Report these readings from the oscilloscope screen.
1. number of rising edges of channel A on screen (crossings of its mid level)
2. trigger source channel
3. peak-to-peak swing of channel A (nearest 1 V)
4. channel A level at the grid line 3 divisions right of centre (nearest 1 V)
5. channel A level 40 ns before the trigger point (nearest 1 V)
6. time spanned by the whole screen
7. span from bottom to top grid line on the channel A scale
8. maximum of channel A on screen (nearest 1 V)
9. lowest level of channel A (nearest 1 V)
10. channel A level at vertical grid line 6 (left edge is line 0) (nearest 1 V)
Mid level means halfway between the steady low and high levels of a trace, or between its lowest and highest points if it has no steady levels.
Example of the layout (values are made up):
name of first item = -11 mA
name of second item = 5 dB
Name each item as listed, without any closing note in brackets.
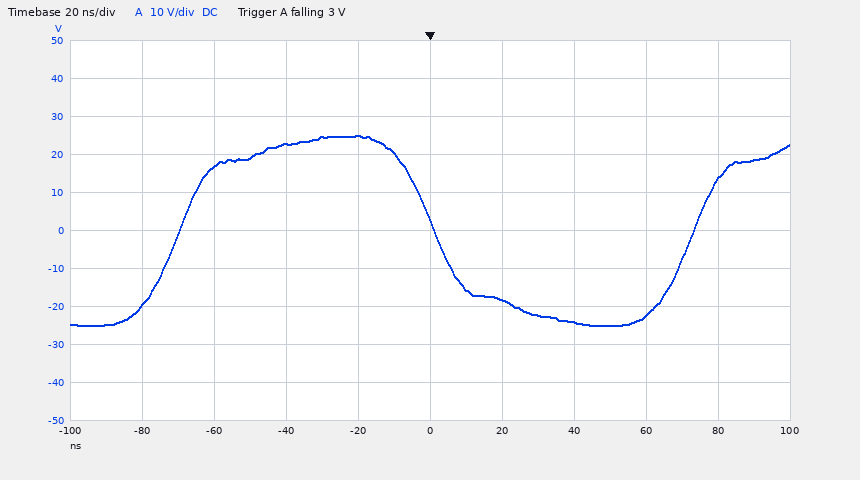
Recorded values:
number of rising edges of channel A on screen = 2
trigger source channel = channel A
peak-to-peak swing of channel A = 50 V
channel A level at the grid line 3 divisions right of centre = -22 V
channel A level 40 ns before the trigger point = 23 V
time spanned by the whole screen = 200 ns
span from bottom to top grid line on the channel A scale = 100 V
maximum of channel A on screen = 25 V
lowest level of channel A = -25 V
channel A level at vertical grid line 6 (left edge is line 0) = -18 V
